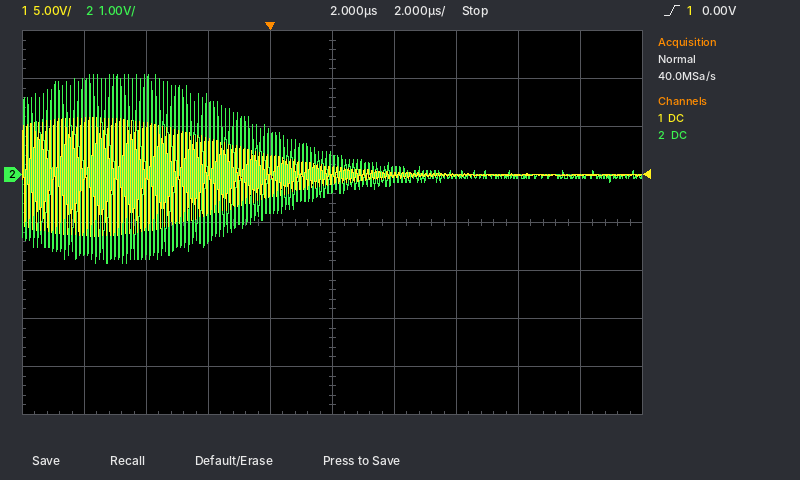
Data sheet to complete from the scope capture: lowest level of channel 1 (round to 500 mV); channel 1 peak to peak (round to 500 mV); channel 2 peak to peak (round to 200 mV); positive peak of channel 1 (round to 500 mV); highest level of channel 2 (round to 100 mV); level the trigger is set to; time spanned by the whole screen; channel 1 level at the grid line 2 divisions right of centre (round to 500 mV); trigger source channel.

-6.5 V
12.5 V
4.0 V
6.0 V
2.1 V
0.00 V
20 µs
0.0 V
channel 1
